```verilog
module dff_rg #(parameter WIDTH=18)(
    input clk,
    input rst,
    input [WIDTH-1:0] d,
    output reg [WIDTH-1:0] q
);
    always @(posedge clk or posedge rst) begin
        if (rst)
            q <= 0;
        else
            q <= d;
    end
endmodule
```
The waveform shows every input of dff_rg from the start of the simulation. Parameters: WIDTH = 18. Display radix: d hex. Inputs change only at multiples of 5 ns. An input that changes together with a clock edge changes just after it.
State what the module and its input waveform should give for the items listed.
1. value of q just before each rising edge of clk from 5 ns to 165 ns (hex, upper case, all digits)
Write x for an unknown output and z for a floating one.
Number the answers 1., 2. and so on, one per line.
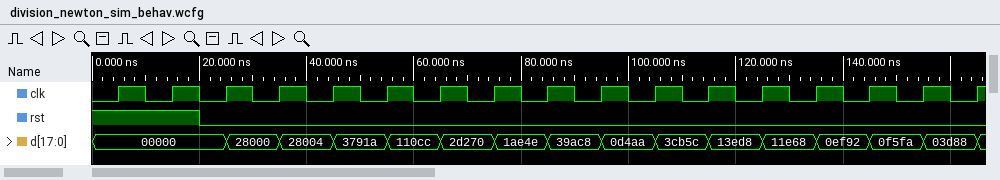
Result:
1. 00000, 00000, 00000, 00000, 28000, 28004, 3791A, 110CC, 2D270, 1AE4E, 39AC8, 0D4AA, 3CB5C, 13ED8, 11E68, 0EF92, 0F5FA
